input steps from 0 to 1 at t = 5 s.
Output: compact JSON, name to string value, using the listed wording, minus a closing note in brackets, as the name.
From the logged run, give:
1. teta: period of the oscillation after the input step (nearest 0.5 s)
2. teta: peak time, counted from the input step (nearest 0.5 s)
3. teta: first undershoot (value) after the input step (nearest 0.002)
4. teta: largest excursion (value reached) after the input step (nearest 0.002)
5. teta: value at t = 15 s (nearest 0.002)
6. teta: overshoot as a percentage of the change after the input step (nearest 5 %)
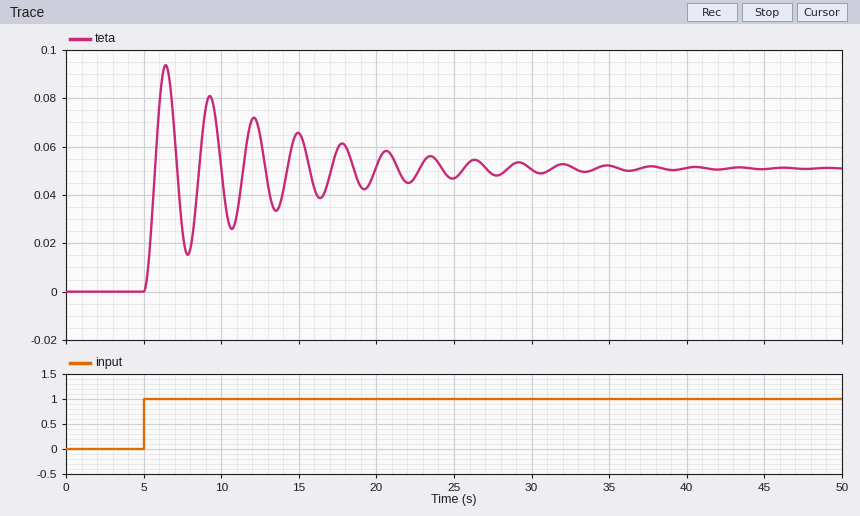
{"teta: period of the oscillation after the input step": "3.0 s", "teta: peak time, counted from the input step": "1.5 s", "teta: first undershoot (value) after the input step": "0.016", "teta: largest excursion (value reached) after the input step": "0.094", "teta: value at t = 15 s": "0.066", "teta: overshoot as a percentage of the change after the input step": "85 %"}
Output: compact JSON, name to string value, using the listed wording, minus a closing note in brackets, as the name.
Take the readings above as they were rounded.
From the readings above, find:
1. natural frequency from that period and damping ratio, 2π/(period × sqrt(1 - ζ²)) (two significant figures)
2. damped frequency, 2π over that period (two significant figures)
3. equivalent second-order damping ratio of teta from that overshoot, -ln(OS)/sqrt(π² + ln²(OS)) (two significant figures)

{"natural frequency from that period and damping ratio, 2π/(period × sqrt(1 - ζ²))": "2.1 rad/s", "damped frequency, 2π over that period": "2.1 rad/s", "equivalent second-order damping ratio of teta from that overshoot, -ln(OS)/sqrt(π² + ln²(OS))": "0.052"}
